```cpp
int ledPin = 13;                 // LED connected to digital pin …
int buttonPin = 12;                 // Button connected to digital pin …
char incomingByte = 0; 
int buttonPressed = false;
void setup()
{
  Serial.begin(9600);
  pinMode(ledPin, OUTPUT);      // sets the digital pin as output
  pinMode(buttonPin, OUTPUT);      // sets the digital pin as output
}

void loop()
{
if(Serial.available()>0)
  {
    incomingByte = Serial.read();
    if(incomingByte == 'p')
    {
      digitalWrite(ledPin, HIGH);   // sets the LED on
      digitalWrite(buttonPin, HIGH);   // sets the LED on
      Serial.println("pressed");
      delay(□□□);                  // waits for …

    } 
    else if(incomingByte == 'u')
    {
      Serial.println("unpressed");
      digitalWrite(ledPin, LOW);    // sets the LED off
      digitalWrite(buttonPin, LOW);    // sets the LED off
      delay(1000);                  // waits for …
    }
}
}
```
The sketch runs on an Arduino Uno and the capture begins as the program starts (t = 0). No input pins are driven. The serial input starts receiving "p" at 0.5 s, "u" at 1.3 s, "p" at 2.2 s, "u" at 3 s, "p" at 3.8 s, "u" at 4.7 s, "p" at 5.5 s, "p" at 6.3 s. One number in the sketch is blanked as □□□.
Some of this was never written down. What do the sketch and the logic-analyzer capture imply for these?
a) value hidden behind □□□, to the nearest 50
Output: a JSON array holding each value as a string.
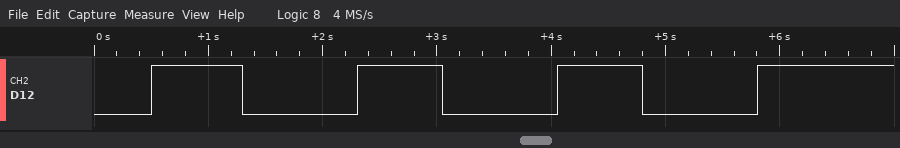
["750"]
